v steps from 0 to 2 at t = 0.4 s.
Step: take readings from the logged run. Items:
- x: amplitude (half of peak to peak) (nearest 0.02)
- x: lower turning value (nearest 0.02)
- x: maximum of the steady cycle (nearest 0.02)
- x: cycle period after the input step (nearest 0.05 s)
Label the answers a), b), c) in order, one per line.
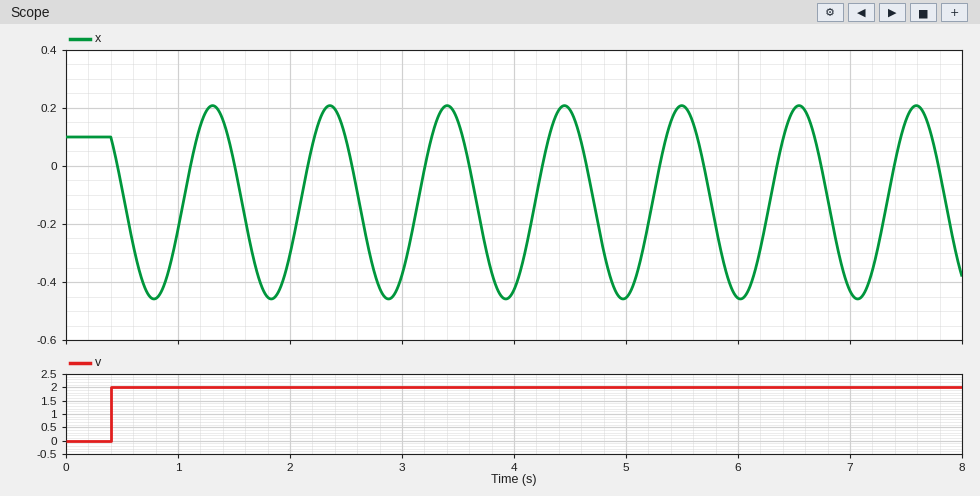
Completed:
a) 0.34
b) -0.46
c) 0.20
d) 1.05 s
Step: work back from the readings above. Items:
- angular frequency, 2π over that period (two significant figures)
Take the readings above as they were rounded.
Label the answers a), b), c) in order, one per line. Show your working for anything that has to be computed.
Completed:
a) 2π / 1.05 = 6.0 rad/s
